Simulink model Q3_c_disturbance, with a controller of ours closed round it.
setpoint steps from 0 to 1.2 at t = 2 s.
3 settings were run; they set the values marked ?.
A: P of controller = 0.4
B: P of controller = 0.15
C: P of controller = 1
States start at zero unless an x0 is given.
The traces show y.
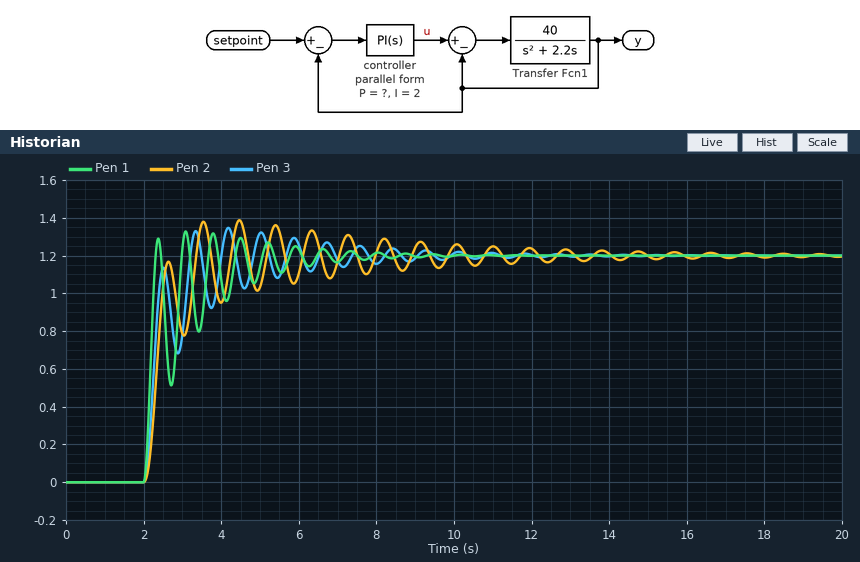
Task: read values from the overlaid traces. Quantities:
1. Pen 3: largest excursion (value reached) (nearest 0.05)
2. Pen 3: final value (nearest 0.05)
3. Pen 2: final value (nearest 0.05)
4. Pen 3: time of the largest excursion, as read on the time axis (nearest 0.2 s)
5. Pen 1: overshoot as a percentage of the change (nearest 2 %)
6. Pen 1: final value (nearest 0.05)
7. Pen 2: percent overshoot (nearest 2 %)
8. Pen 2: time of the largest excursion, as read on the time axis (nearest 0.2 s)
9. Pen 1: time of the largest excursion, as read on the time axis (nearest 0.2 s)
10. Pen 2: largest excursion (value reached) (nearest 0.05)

1.35
1.20
1.20
4.2 s
10 %
1.20
16 %
4.4 s
3.0 s
1.40
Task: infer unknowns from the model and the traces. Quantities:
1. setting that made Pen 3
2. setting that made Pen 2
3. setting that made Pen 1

A
B
C
